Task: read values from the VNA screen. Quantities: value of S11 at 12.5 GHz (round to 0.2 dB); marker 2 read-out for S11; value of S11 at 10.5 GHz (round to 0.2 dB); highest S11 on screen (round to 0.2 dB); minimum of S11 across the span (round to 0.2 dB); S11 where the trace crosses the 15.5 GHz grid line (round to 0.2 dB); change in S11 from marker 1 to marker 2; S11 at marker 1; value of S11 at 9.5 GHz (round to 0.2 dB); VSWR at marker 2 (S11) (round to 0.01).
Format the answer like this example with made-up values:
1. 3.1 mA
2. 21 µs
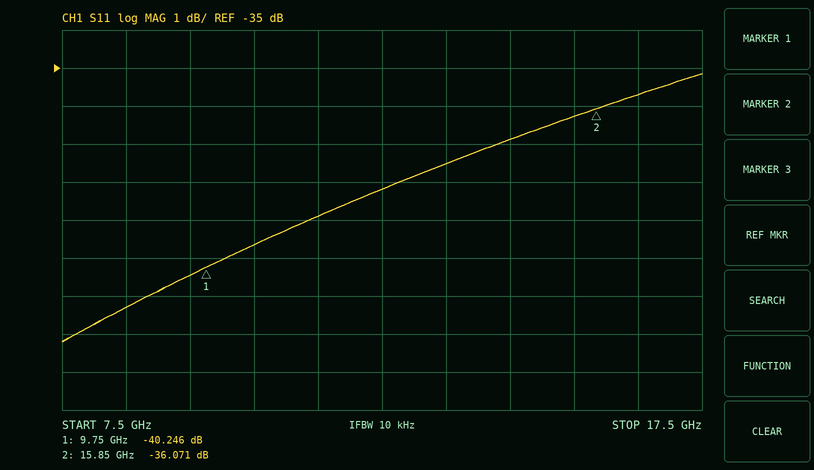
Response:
1. -38.2 dB
2. -36.071 dB
3. -39.6 dB
4. -35.2 dB
5. -42.2 dB
6. -36.2 dB
7. 4.175 dB
8. -40.246 dB
9. -40.4 dB
10. 1.03
